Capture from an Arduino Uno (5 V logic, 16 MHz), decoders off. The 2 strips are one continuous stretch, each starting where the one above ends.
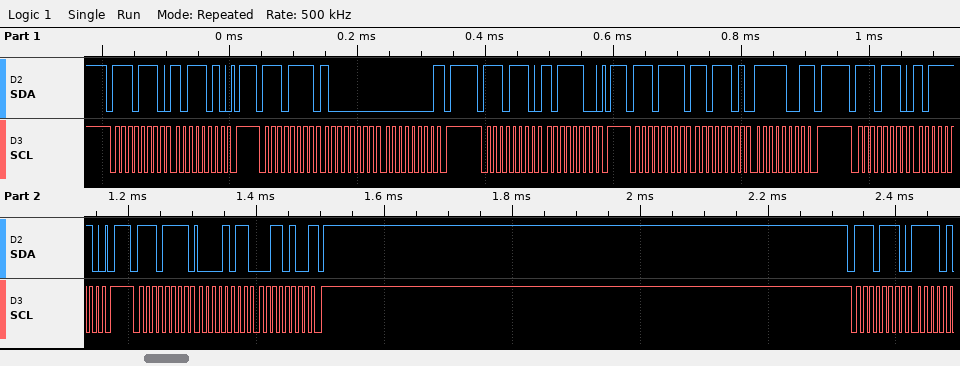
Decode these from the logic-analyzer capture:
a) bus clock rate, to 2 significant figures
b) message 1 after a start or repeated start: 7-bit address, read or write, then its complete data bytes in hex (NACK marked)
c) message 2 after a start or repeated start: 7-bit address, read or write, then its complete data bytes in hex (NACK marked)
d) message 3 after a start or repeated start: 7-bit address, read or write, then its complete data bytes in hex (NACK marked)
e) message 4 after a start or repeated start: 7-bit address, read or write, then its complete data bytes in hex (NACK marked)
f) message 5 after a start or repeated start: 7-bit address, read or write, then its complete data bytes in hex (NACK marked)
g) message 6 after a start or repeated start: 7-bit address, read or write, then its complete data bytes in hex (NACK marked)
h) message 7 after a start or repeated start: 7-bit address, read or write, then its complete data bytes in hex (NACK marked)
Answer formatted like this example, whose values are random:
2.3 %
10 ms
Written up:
100 kHz
0x77 write: BA
0x77 read: 80 00 NACK
0x77 write: BC
0x77 read: DD F9 NACK
0x77 write: BE
0x77 read: 0B 34 NACK
0x77 write
